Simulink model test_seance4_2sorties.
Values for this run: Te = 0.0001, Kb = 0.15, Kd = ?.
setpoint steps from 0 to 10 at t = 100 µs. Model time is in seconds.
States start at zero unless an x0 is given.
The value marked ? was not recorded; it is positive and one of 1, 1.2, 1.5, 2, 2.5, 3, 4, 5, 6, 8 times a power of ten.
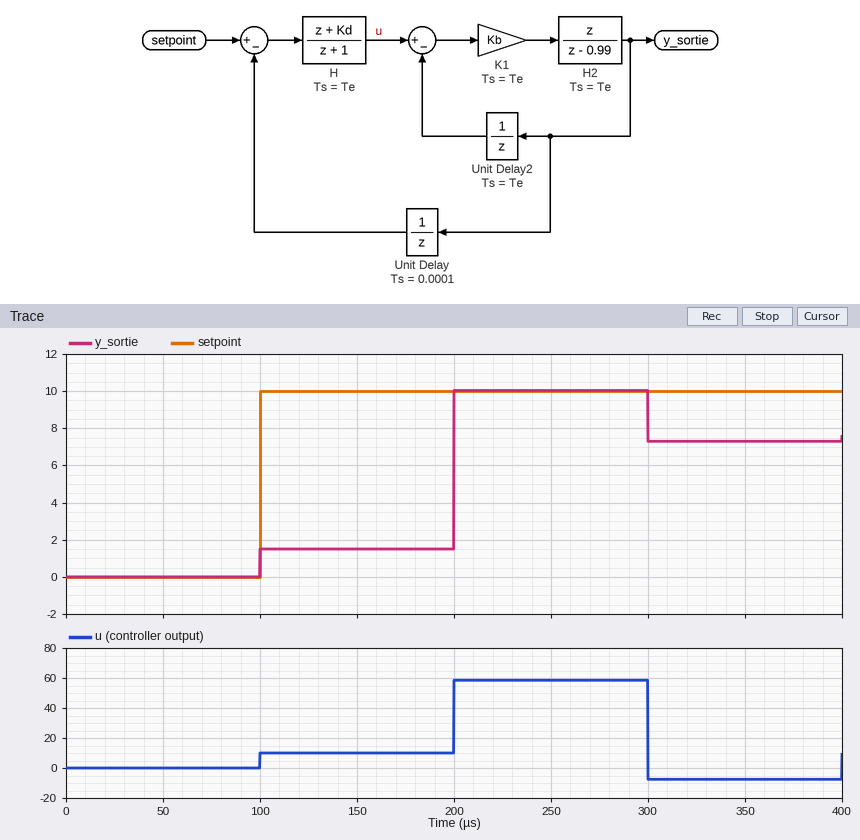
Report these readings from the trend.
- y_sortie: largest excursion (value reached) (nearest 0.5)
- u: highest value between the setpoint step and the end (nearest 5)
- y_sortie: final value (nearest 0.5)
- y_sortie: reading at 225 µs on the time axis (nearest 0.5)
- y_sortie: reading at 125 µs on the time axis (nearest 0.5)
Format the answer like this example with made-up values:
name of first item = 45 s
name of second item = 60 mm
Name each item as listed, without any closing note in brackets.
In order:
y_sortie: largest excursion (value reached) = 10.0
u: highest value between the setpoint step and the end = 60
y_sortie: final value = 7.5
y_sortie: reading at 225 µs on the time axis = 10.0
y_sortie: reading at 125 µs on the time axis = 1.5
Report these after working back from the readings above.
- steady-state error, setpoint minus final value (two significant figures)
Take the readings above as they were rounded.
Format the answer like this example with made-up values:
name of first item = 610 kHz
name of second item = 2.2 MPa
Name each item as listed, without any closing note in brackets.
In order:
steady-state error, setpoint minus final value = 2.5
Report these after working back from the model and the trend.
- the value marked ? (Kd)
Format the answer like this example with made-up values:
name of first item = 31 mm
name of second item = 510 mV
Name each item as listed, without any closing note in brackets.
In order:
the value marked ? = 6
